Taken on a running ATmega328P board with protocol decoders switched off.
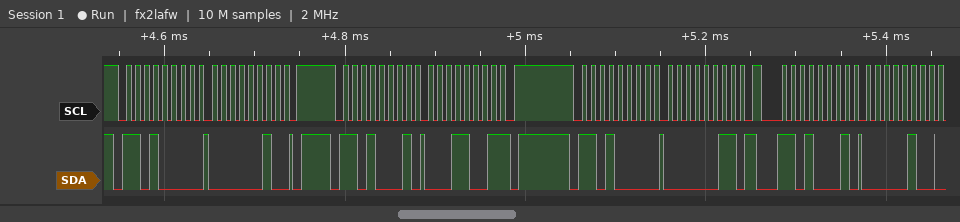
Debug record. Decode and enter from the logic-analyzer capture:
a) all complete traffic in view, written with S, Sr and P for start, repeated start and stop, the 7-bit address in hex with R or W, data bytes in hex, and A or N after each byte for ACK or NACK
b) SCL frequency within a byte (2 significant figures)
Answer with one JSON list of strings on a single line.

["S 68W A 02 A P S 68R A 19 N P S 68W A 03 A Sr 68R A 04 A", "100 kHz"]
